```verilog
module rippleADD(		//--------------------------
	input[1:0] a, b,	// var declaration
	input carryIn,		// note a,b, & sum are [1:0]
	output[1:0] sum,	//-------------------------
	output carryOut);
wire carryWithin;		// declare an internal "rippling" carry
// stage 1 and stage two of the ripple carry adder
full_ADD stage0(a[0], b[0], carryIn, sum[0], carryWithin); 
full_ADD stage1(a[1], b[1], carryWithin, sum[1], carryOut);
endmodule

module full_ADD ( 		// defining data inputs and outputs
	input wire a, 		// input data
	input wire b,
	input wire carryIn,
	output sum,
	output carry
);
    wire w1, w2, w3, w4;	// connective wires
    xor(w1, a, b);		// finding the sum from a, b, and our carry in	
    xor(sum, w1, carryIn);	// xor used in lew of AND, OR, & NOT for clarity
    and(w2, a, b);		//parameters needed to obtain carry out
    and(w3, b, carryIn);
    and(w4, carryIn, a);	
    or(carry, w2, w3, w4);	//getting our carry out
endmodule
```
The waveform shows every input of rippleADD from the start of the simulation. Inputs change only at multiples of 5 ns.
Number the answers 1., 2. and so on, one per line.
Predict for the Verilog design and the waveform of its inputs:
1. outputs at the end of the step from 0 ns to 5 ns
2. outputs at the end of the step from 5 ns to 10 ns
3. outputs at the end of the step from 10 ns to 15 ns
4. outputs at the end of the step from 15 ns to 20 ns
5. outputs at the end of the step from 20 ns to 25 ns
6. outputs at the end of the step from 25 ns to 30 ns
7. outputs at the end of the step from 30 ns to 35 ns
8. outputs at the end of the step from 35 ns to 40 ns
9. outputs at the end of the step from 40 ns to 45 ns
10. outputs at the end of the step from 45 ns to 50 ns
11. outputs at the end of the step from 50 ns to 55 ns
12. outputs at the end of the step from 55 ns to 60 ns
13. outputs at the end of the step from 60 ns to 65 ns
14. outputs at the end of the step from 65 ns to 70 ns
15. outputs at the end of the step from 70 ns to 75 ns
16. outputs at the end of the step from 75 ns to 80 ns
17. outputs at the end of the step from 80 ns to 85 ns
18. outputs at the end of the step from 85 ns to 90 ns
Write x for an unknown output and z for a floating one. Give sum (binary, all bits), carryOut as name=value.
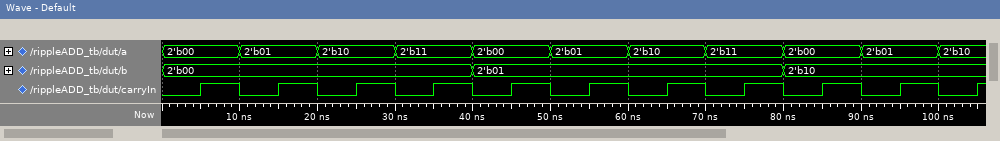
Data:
1. sum=00, carryOut=0
2. sum=01, carryOut=0
3. sum=01, carryOut=0
4. sum=10, carryOut=0
5. sum=10, carryOut=0
6. sum=11, carryOut=0
7. sum=11, carryOut=0
8. sum=00, carryOut=1
9. sum=01, carryOut=0
10. sum=10, carryOut=0
11. sum=10, carryOut=0
12. sum=11, carryOut=0
13. sum=11, carryOut=0
14. sum=00, carryOut=1
15. sum=00, carryOut=1
16. sum=01, carryOut=1
17. sum=10, carryOut=0
18. sum=11, carryOut=0
